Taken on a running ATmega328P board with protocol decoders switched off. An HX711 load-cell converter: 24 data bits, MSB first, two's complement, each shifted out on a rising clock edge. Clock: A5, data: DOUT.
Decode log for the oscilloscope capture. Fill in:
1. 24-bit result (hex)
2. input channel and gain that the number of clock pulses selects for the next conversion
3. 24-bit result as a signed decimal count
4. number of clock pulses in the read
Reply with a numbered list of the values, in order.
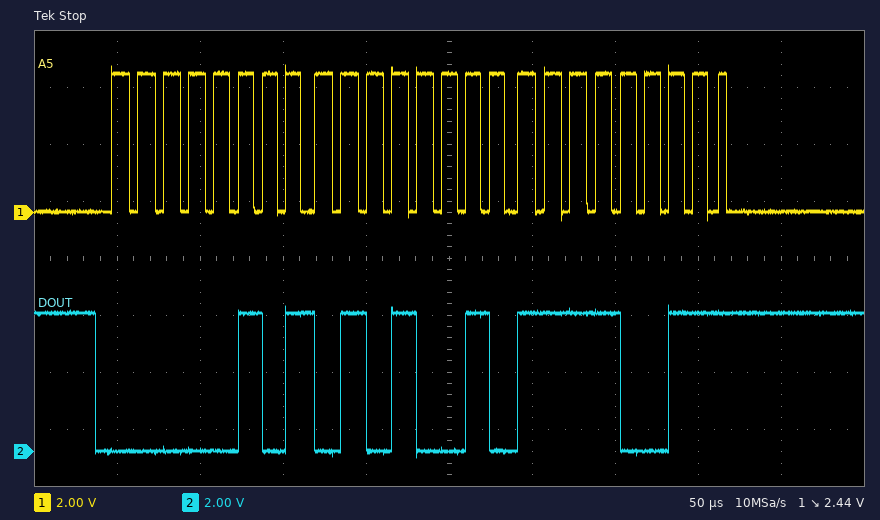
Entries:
1. 0x0552F3
2. channel A, gain 128
3. 348915
4. 25
